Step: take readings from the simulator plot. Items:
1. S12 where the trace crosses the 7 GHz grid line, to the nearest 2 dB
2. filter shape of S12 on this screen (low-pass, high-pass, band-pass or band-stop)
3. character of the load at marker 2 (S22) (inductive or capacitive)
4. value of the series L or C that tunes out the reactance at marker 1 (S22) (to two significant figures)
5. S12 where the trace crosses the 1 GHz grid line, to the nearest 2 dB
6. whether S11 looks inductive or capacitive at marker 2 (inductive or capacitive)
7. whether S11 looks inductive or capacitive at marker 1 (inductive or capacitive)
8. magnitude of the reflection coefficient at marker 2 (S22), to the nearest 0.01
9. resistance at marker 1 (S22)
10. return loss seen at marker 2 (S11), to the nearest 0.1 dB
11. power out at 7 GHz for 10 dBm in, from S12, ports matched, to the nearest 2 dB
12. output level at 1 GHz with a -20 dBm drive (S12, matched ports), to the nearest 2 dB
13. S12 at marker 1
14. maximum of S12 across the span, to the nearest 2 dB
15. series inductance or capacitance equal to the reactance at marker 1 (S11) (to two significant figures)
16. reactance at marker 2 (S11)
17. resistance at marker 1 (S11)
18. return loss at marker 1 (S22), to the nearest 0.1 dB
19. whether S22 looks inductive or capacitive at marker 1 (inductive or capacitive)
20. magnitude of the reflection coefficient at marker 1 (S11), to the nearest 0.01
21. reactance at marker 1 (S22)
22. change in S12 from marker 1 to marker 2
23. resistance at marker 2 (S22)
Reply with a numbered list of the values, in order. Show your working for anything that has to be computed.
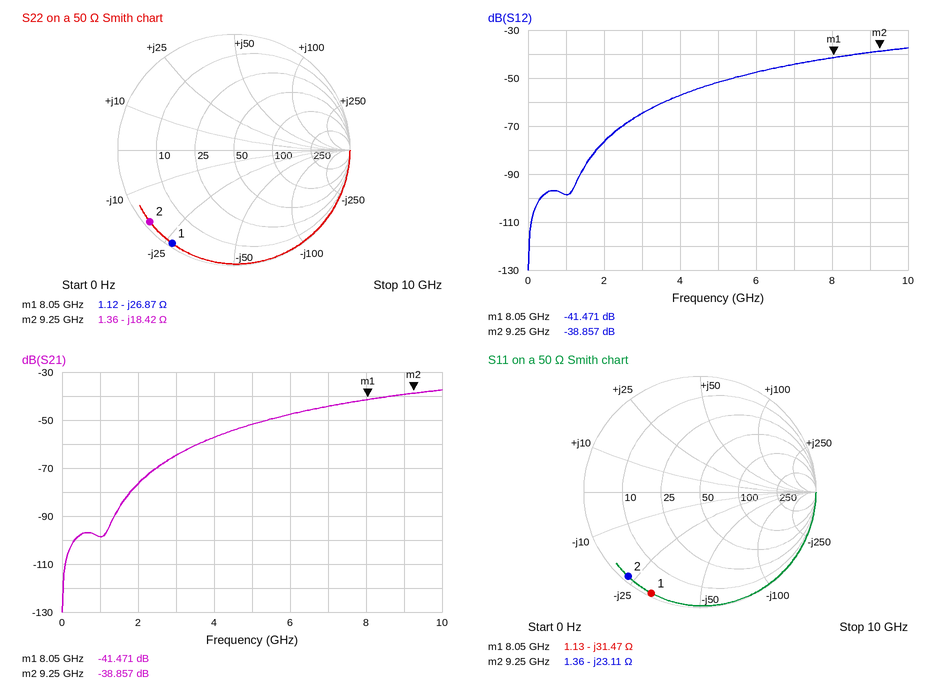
1. -44 dB
2. high-pass
3. capacitive
4. L = 26.87 Ω/(2π × 8.05 GHz) ≈ 531 pH, so 530 pH to two significant figures
5. -98 dB
6. capacitive
7. capacitive
8. 0.95
9. 1.12 Ω
10. 0.4 dB
11. 10 dBm + (-44 dB) = -34 dBm
12. -20 dBm + (-98 dB) = -118 dBm
13. -41.471 dB
14. -38 dB
15. C = 1/(2π × 8.05 GHz × 31.47 Ω) ≈ 628 fF, so 630 fF to two significant figures
16. -23.11 Ω
17. 1.13 Ω
18. 0.3 dB
19. capacitive
20. 0.97
21. -26.87 Ω
22. -38.857 − (-41.471) = 2.614 dB
23. 1.36 Ω
